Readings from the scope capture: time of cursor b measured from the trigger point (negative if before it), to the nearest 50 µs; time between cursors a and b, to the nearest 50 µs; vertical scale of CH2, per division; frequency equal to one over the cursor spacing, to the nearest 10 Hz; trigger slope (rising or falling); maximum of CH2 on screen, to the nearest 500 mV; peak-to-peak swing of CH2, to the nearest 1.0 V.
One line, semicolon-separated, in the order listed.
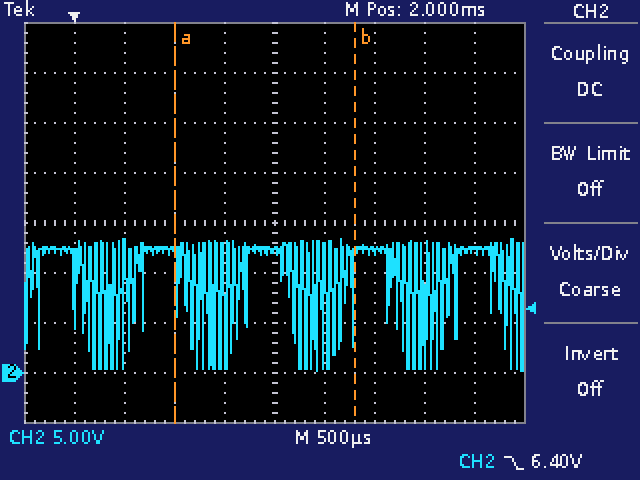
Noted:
+2.80 ms; 1.80 ms; 5 V; 560 Hz; falling; 13.5 V; 13.0 V
